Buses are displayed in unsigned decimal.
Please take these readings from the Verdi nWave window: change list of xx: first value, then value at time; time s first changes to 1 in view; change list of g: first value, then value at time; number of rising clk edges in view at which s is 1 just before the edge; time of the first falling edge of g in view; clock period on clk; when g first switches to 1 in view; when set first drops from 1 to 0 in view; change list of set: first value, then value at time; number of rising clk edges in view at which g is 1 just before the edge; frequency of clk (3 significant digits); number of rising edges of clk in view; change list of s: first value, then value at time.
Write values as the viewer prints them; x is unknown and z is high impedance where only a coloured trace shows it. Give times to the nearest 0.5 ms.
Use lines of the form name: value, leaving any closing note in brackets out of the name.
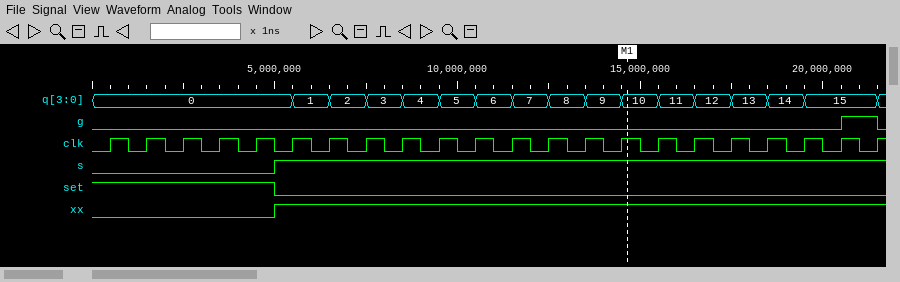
change list of xx: first value, then value at time: 0, 1 at 5 ms
time s first changes to 1 in view: 5 ms
change list of g: first value, then value at time: 0, 1 at 20.5 ms, 0 at 21.5 ms
number of rising clk edges in view at which s is 1 just before the edge: 17
time of the first falling edge of g in view: 21.5 ms
clock period on clk: 1 ms
when g first switches to 1 in view: 20.5 ms
when set first drops from 1 to 0 in view: 5 ms
change list of set: first value, then value at time: 1, 0 at 5 ms
number of rising clk edges in view at which g is 1 just before the edge: 1
frequency of clk: 1.00 kHz
number of rising edges of clk in view: 22
change list of s: first value, then value at time: 0, 1 at 5 ms
